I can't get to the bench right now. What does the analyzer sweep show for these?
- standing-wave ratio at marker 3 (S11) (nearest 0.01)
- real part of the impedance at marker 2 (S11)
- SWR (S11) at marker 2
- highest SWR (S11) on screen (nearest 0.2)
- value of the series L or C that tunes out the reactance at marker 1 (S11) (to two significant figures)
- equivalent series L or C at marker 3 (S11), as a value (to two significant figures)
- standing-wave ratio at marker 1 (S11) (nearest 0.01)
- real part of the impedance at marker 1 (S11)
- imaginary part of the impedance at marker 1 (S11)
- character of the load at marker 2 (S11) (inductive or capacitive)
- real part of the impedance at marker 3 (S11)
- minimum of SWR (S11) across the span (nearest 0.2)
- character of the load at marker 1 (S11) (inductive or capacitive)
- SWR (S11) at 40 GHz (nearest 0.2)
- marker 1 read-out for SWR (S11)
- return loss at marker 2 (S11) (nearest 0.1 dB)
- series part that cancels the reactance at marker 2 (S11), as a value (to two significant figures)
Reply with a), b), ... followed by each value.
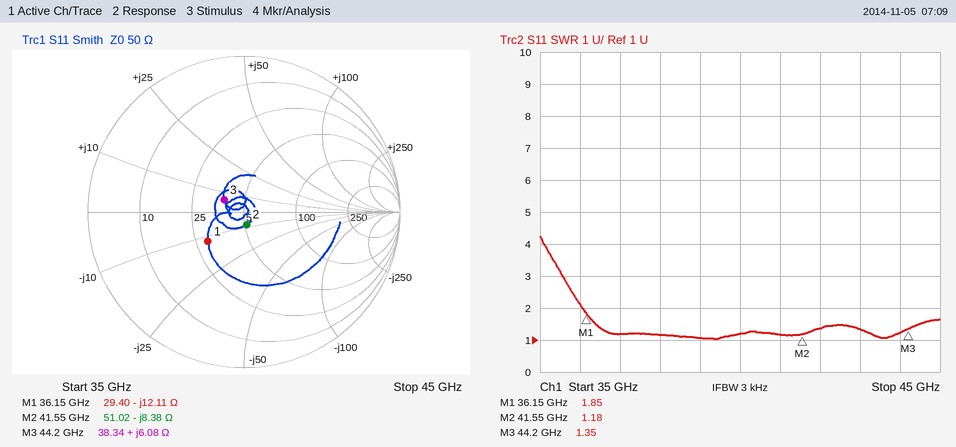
a) 1.35
b) 51.02 Ω
c) 1.18
d) 4.2
e) 53 pH
f) 22 pH
g) 1.85
h) 29.40 Ω
i) -12.11 Ω
j) capacitive
k) 38.34 Ω
l) 1.0
m) capacitive
n) 1.2
o) 1.85
p) 21.6 dB
q) 32 pH
